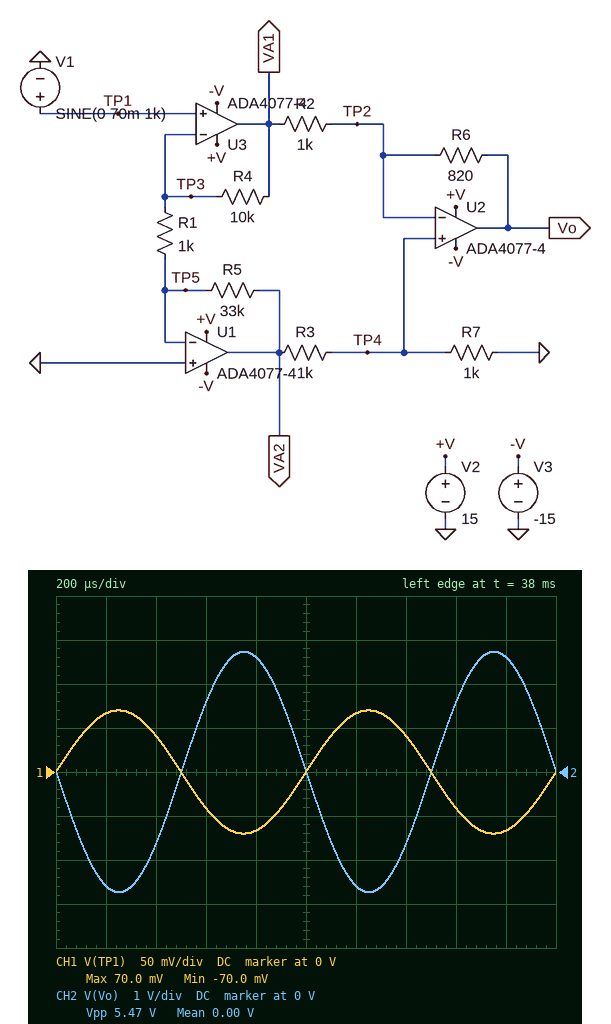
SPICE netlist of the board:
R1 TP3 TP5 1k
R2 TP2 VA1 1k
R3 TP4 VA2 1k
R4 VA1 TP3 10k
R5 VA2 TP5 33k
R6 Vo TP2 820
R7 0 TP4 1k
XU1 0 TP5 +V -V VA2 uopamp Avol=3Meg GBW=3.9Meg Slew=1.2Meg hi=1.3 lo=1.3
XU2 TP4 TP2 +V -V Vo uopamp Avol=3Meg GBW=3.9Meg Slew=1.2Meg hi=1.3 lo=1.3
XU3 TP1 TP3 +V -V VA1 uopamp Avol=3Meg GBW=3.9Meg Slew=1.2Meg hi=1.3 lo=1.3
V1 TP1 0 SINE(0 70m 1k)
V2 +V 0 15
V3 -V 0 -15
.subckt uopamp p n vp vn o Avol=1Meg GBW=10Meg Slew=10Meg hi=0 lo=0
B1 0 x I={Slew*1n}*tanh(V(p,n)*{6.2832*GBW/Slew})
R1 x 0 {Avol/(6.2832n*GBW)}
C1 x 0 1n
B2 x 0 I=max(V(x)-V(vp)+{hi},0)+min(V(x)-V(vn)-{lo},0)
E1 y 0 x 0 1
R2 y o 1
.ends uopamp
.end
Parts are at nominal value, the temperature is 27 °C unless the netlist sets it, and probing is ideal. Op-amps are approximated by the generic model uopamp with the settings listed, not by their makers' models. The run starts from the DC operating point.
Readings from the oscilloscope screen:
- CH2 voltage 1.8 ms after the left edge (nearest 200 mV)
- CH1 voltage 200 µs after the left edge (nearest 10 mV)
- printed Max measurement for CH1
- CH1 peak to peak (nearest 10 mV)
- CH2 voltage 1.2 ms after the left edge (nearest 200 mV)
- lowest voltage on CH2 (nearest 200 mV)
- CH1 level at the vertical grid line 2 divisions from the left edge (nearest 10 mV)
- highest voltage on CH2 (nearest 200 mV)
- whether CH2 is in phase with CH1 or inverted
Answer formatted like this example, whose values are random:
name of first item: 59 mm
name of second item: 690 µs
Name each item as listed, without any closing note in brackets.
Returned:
CH2 voltage 1.8 ms after the left edge: 2.6 V
CH1 voltage 200 µs after the left edge: 70 mV
printed Max measurement for CH1: 70.0 mV
CH1 peak to peak: 140 mV
CH2 voltage 1.2 ms after the left edge: -2.6 V
lowest voltage on CH2: -2.8 V
CH1 level at the vertical grid line 2 divisions from the left edge: 40 mV
highest voltage on CH2: 2.8 V
whether CH2 is in phase with CH1 or inverted: inverted
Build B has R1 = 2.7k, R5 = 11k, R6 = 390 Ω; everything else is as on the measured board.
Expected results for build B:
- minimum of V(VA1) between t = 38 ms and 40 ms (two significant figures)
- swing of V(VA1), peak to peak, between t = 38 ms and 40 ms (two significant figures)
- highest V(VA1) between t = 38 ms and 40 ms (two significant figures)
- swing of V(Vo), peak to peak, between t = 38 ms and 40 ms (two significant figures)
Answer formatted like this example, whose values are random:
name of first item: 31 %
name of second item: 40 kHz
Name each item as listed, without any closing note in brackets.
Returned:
minimum of V(VA1) between t = 38 ms and 40 ms: -330 mV
swing of V(VA1), peak to peak, between t = 38 ms and 40 ms: 660 mV
highest V(VA1) between t = 38 ms and 40 ms: 330 mV
swing of V(Vo), peak to peak, between t = 38 ms and 40 ms: 650 mV
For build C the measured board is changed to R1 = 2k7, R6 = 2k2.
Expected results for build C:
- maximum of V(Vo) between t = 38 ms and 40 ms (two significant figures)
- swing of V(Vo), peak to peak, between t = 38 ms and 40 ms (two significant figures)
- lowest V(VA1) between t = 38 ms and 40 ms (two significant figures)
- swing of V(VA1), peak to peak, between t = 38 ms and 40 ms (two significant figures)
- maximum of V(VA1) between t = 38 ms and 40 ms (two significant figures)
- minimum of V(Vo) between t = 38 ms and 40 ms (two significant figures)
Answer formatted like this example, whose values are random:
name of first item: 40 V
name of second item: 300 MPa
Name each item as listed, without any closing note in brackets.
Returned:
maximum of V(Vo) between t = 38 ms and 40 ms: 2.1 V
swing of V(Vo), peak to peak, between t = 38 ms and 40 ms: 4.2 V
lowest V(VA1) between t = 38 ms and 40 ms: -330 mV
swing of V(VA1), peak to peak, between t = 38 ms and 40 ms: 660 mV
maximum of V(VA1) between t = 38 ms and 40 ms: 330 mV
minimum of V(Vo) between t = 38 ms and 40 ms: -2.1 V
